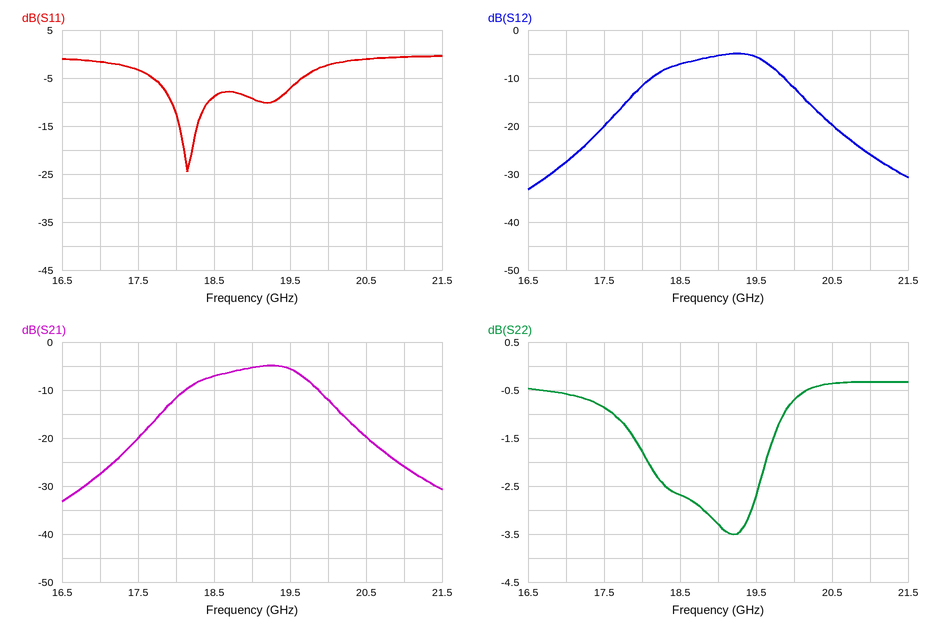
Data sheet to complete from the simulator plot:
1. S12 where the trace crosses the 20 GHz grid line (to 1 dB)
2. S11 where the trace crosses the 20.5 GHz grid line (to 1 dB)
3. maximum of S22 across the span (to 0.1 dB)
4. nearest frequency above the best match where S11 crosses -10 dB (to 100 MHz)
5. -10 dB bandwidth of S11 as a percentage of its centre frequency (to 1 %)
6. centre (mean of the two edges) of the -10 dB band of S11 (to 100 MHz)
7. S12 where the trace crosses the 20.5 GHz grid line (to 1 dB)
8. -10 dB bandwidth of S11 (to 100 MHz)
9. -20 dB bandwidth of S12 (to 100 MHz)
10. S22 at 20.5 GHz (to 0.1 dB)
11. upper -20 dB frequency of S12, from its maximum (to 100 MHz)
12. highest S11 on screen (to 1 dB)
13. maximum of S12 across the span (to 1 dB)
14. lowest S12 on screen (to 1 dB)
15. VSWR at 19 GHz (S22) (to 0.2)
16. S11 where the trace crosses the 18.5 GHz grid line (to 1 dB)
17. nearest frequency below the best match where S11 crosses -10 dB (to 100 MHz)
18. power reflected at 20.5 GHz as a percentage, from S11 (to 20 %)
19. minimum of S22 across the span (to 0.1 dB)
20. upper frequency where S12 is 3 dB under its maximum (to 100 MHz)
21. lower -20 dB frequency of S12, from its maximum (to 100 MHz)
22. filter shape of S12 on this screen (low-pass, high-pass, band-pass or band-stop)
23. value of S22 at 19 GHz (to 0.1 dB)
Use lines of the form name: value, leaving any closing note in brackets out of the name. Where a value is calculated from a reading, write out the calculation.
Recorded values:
S12 where the trace crosses the 20 GHz grid line: -12 dB
S11 where the trace crosses the 20.5 GHz grid line: -1 dB
maximum of S22 across the span: -0.3 dB
nearest frequency above the best match where S11 crosses -10 dB: 18.4 GHz
-10 dB bandwidth of S11 as a percentage of its centre frequency: 500 MHz / 18.15 GHz ≈ 3 %
centre (mean of the two edges) of the -10 dB band of S11: 18.2 GHz
S12 where the trace crosses the 20.5 GHz grid line: -20 dB
-10 dB bandwidth of S11: 18.4 GHz − 17.9 GHz = 500 MHz
-20 dB bandwidth of S12: 20.9 GHz − 17.2 GHz = 3.7 GHz
S22 at 20.5 GHz: -0.4 dB
upper -20 dB frequency of S12, from its maximum: 20.9 GHz
highest S11 on screen: 0 dB
maximum of S12 across the span: -5 dB
lowest S12 on screen: -33 dB
VSWR at 19 GHz (S22): |Γ| = 10^(-3.3/20) = 0.6839; VSWR = (1 + 0.6839)/(1 − 0.6839) ≈ 5.33, so 5.4 to the nearest 0.2
S11 where the trace crosses the 18.5 GHz grid line: -9 dB
nearest frequency below the best match where S11 crosses -10 dB: 17.9 GHz
power reflected at 20.5 GHz as a percentage, from S11: 10^(-1/10) ≈ 79.4 %, so 80 % to the nearest 20 %
minimum of S22 across the span: -3.5 dB
upper frequency where S12 is 3 dB under its maximum: 19.7 GHz
lower -20 dB frequency of S12, from its maximum: 17.2 GHz
filter shape of S12 on this screen: band-pass
value of S22 at 19 GHz: -3.3 dB
